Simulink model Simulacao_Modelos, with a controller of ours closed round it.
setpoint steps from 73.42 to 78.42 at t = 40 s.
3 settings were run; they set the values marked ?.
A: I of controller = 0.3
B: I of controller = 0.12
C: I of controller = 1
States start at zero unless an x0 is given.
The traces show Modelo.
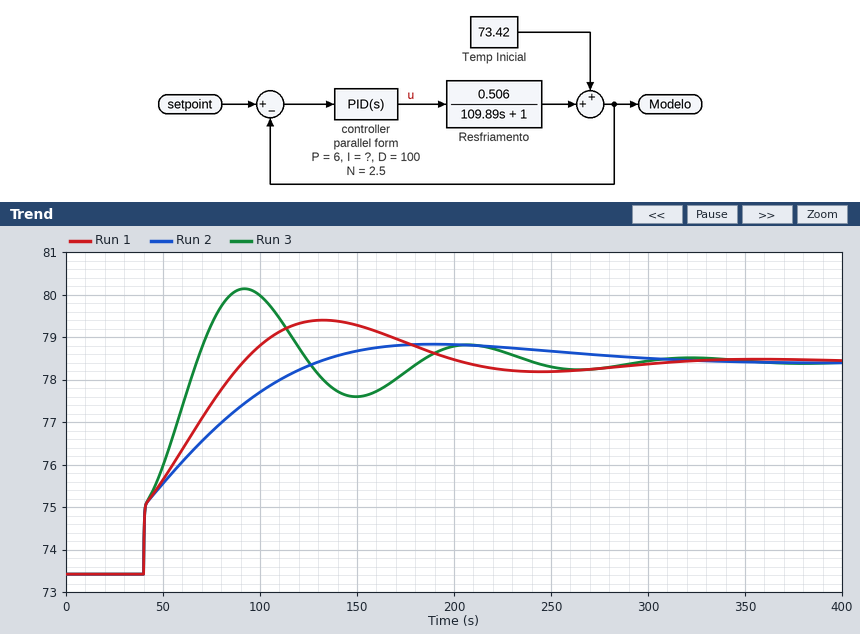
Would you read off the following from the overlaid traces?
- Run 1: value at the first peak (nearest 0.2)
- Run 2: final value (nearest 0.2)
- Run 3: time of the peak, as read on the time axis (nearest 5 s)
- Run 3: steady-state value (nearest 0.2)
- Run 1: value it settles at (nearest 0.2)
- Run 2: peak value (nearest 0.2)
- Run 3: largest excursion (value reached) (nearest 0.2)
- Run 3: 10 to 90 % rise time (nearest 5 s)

79.4
78.4
90 s
78.4
78.4
78.8
80.2
25 s
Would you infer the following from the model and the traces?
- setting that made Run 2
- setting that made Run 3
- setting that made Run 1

B
C
A
